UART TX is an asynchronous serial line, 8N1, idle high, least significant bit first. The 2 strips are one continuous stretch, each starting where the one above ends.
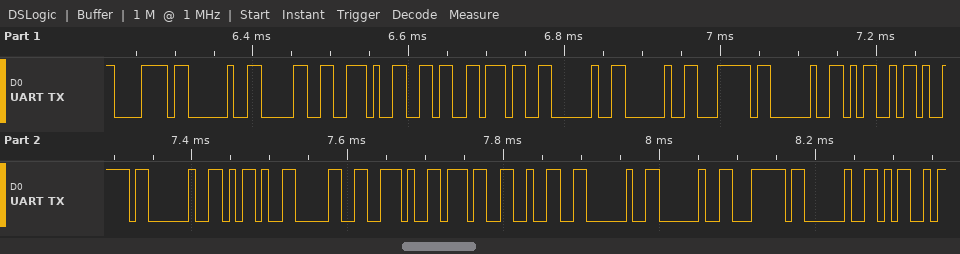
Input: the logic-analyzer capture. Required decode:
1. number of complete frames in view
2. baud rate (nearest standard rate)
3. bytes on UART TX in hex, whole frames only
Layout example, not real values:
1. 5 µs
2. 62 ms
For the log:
1. 23
2. 115200 baud
3. 78 20 30 2E 36 37 20 20 7C 20 4D 79 20 2D 30 2E 37 32 20 20 7C 20 4D
